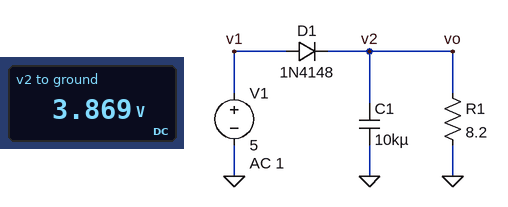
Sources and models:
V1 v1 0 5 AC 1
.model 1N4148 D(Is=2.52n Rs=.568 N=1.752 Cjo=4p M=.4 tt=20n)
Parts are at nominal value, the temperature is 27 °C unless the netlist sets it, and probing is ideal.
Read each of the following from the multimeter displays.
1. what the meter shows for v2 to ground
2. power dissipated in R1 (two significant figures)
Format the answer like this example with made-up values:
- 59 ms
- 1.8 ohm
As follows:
- 3.869 V
- 1.8 W
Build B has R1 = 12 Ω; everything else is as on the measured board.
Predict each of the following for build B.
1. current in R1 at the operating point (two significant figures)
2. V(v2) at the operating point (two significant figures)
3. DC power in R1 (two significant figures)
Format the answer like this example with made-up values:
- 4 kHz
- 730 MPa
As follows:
- 330 mA
- 4.0 V
- 1.3 W
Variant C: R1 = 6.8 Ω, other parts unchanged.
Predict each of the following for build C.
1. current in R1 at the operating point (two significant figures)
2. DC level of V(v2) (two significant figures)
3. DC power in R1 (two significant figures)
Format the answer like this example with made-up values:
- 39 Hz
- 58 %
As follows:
- 560 mA
- 3.8 V
- 2.1 W
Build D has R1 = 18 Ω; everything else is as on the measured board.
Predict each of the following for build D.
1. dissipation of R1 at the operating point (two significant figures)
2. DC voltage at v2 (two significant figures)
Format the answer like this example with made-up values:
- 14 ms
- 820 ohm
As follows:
- 910 mW
- 4.0 V
